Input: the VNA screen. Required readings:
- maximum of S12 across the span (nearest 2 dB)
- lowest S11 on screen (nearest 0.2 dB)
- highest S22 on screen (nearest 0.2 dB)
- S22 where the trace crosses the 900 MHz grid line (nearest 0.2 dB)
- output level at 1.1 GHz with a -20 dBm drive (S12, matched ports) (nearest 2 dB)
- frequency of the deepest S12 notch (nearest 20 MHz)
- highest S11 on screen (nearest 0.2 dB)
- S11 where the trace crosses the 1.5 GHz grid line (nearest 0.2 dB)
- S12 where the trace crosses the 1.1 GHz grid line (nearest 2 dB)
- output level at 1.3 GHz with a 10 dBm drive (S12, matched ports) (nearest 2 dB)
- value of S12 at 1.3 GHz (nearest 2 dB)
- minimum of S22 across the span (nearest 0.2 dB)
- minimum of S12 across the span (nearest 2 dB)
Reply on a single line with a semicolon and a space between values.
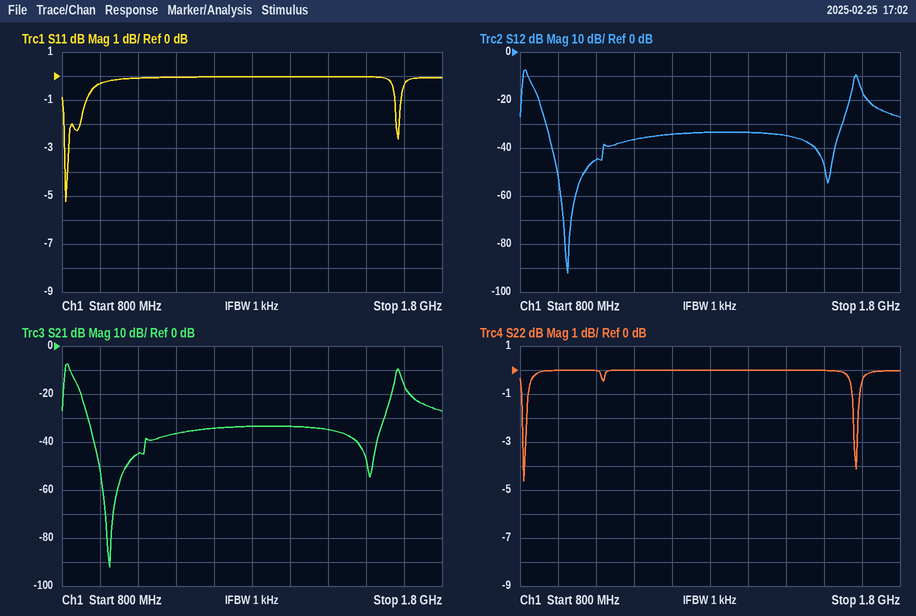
-8 dB; -5.2 dB; 0.0 dB; 0.0 dB; -56 dBm; 920 MHz; 0.0 dB; 0.0 dB; -36 dB; -24 dBm; -34 dB; -4.6 dB; -92 dB
